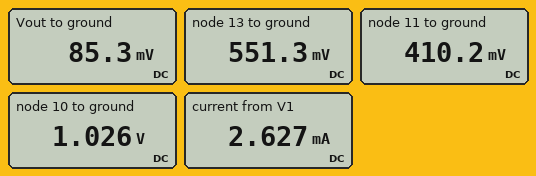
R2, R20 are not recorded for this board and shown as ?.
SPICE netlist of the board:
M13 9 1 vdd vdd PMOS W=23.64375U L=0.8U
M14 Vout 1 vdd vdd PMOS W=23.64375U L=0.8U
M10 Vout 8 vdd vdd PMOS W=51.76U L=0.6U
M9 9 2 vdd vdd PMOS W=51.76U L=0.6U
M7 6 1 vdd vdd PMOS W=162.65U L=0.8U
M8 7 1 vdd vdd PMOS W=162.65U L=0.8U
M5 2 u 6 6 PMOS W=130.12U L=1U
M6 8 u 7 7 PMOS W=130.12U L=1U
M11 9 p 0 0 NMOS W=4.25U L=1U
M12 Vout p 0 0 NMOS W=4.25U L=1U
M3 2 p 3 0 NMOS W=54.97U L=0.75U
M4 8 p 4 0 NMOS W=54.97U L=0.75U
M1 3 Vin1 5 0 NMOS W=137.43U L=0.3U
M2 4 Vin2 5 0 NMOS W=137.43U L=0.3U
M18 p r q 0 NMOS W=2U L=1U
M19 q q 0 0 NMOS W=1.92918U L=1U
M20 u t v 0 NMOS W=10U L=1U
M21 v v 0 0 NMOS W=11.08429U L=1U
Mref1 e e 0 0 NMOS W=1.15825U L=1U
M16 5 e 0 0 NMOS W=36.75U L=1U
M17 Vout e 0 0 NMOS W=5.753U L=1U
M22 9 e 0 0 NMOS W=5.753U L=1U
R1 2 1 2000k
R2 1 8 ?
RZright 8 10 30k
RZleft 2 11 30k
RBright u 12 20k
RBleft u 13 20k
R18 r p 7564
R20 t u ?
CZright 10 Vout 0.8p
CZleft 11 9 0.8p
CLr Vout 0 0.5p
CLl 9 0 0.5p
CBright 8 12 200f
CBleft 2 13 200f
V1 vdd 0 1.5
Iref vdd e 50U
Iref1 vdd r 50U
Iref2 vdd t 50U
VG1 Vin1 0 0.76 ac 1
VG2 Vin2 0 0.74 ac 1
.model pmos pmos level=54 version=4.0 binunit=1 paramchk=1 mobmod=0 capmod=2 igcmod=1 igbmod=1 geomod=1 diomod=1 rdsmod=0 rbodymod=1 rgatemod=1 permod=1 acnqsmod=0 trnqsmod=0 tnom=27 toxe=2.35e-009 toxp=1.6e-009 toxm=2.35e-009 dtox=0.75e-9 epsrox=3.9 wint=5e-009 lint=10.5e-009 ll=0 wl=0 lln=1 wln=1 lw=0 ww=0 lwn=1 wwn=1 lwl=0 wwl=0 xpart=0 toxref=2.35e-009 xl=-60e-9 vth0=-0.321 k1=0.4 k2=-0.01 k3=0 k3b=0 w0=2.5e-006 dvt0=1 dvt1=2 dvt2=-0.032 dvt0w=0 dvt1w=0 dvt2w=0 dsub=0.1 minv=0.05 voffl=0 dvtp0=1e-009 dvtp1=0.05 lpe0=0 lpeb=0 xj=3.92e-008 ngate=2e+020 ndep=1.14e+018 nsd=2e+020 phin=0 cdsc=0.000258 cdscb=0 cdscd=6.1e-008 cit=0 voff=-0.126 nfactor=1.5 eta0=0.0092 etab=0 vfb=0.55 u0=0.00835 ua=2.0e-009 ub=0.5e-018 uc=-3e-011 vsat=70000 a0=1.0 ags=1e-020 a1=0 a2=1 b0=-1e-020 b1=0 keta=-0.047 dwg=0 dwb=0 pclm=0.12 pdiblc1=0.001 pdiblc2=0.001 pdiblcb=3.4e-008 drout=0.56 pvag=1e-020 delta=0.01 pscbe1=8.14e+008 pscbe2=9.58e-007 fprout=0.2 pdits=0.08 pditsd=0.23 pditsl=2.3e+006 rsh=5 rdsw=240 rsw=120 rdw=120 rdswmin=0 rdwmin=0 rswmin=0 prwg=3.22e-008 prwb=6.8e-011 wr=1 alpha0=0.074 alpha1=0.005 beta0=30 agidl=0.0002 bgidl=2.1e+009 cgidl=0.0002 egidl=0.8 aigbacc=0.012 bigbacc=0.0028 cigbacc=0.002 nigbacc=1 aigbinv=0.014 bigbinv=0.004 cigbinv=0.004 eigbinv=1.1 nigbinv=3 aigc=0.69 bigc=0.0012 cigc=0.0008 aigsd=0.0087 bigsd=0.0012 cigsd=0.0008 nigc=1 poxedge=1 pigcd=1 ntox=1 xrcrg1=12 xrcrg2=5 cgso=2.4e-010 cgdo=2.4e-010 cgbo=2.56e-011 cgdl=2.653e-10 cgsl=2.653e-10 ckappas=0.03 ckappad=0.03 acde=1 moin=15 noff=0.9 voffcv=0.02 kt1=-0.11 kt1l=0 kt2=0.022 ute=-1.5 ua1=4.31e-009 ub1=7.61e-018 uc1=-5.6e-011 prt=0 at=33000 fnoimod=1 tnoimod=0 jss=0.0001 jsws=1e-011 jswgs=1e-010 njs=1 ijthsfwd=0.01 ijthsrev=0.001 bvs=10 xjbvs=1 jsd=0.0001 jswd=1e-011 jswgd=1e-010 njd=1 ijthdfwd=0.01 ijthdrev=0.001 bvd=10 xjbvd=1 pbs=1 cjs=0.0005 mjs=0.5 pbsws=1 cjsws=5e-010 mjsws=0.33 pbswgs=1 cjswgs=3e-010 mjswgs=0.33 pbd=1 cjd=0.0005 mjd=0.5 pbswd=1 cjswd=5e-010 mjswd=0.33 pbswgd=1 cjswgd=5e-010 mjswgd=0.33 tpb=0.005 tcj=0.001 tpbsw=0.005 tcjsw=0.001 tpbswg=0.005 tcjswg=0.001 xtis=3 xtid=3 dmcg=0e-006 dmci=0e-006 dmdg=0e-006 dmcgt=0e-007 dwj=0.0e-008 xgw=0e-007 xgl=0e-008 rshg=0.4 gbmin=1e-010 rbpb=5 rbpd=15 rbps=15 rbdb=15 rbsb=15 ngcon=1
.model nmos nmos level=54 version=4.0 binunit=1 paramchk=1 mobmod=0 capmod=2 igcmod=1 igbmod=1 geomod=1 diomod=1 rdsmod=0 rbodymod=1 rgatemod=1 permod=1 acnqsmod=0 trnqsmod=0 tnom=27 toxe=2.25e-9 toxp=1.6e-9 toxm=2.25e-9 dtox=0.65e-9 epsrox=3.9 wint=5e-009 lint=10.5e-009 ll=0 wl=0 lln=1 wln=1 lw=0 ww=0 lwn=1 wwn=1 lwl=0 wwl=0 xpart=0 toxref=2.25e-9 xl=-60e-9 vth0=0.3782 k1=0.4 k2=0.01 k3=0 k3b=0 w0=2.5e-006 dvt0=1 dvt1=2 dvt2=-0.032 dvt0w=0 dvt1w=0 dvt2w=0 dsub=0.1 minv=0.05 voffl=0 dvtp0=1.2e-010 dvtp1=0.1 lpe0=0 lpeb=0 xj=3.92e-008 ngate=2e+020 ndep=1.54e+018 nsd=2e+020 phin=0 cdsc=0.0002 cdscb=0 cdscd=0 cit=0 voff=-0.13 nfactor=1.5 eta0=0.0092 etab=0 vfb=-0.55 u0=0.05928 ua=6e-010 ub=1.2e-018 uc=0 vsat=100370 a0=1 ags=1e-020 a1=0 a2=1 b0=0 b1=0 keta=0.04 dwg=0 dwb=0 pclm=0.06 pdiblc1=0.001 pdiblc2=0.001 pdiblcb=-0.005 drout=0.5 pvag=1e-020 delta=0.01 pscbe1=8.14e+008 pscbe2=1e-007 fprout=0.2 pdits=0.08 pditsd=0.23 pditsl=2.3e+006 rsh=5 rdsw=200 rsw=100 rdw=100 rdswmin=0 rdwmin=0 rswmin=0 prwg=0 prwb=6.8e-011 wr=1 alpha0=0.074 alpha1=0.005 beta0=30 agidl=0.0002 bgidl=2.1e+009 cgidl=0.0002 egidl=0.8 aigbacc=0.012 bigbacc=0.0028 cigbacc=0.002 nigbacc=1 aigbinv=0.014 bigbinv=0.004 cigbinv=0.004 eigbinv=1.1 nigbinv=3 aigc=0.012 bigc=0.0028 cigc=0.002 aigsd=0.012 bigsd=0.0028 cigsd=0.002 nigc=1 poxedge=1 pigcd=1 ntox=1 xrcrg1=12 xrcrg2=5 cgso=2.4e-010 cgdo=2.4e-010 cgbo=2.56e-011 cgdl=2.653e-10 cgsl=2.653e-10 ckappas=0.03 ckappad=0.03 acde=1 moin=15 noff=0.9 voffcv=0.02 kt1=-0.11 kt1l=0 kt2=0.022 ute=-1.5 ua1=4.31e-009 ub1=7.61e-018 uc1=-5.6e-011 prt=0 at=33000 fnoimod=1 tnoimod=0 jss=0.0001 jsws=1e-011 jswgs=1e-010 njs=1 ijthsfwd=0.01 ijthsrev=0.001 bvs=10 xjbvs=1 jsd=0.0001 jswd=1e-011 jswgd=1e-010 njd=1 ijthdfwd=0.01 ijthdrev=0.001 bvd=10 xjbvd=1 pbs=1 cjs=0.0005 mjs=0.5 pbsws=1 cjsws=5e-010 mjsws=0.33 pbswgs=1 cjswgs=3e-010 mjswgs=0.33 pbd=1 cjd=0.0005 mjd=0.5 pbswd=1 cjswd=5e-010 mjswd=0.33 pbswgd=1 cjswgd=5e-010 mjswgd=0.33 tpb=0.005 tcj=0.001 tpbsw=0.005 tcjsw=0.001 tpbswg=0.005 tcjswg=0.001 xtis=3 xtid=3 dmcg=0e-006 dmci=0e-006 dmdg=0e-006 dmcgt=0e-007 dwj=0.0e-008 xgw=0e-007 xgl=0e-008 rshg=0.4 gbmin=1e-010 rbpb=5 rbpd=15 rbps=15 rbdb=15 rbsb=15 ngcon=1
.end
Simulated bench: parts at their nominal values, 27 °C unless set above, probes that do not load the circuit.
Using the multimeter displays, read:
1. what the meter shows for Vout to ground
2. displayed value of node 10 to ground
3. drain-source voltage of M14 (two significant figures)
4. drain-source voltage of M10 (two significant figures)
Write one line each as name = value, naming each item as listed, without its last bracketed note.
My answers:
what the meter shows for Vout to ground = 85.3 mV
displayed value of node 10 to ground = 1.026 V
drain-source voltage of M14 = -1.4 V
drain-source voltage of M10 = -1.4 V
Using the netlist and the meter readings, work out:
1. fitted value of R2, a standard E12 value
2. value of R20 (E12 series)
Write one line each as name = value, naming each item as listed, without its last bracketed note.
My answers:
fitted value of R2, a standard E12 value = 680 kΩ
value of R20 = 10 kΩ
